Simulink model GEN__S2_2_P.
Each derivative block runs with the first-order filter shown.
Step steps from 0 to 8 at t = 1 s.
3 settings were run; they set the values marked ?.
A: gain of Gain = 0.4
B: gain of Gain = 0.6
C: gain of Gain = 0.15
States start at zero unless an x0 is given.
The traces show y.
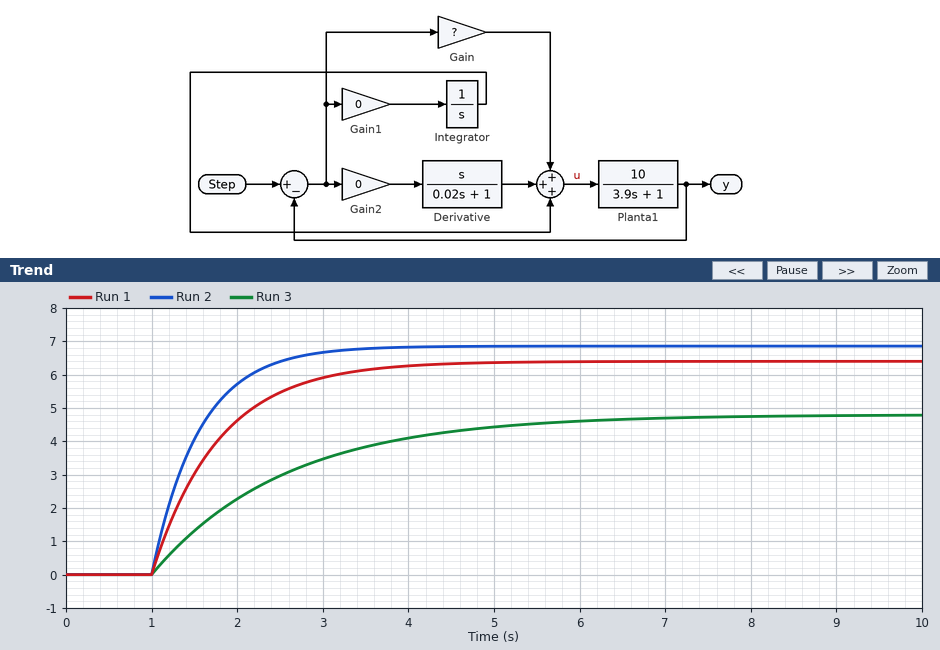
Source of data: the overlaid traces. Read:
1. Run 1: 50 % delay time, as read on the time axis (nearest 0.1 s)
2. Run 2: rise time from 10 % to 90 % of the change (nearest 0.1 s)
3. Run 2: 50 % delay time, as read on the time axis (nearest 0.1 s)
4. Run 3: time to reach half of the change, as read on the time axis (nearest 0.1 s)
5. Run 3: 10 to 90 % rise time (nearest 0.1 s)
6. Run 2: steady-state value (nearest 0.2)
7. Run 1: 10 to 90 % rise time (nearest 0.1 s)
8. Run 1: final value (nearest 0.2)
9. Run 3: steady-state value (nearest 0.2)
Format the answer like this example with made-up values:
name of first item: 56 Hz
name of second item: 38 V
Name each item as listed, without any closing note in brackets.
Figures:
Run 1: 50 % delay time, as read on the time axis: 1.5 s
Run 2: rise time from 10 % to 90 % of the change: 1.2 s
Run 2: 50 % delay time, as read on the time axis: 1.4 s
Run 3: time to reach half of the change, as read on the time axis: 2.1 s
Run 3: 10 to 90 % rise time: 3.4 s
Run 2: steady-state value: 6.8
Run 1: 10 to 90 % rise time: 1.7 s
Run 1: final value: 6.4
Run 3: steady-state value: 4.8
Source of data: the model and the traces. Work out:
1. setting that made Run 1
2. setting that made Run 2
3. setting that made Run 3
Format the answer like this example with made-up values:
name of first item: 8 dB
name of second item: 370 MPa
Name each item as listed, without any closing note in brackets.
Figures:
setting that made Run 1: A
setting that made Run 2: B
setting that made Run 3: C
